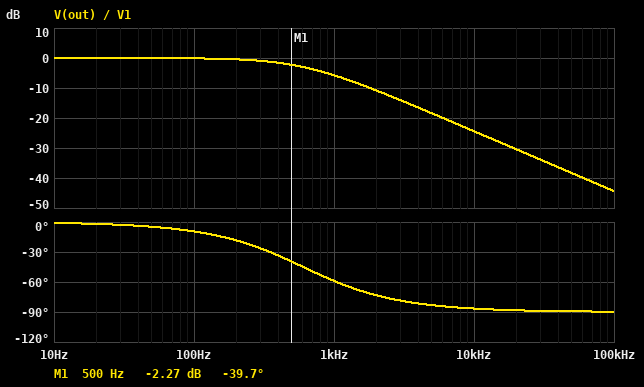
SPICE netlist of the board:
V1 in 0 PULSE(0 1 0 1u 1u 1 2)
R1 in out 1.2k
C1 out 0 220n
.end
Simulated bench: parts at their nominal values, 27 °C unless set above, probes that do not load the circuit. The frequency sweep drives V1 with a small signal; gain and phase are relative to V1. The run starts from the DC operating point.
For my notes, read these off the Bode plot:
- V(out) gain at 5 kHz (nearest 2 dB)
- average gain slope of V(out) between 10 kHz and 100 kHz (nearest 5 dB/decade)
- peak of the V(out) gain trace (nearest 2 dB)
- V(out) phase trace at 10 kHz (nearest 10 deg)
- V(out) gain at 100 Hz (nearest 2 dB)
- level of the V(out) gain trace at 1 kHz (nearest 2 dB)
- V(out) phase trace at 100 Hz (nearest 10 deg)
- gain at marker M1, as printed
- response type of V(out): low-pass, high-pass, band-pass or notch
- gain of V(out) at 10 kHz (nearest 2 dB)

-18 dB
-20 dB/decade
0 dB
-90 deg
0 dB
-6 dB
-10 deg
-2.27 dB
low-pass
-24 dB
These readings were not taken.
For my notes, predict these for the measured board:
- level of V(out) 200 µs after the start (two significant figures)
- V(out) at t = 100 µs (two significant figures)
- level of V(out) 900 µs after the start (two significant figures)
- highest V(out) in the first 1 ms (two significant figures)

530 mV
310 mV
970 mV
980 mV
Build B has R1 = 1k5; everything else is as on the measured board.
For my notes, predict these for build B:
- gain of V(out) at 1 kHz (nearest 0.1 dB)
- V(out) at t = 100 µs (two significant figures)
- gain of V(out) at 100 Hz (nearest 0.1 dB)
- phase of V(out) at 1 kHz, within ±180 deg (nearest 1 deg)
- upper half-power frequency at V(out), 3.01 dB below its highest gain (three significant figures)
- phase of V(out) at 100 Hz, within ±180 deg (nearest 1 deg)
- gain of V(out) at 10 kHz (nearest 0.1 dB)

-7.2 dB
260 mV
-0.2 dB
-64 deg
482 Hz
-12 deg
-26.3 dB
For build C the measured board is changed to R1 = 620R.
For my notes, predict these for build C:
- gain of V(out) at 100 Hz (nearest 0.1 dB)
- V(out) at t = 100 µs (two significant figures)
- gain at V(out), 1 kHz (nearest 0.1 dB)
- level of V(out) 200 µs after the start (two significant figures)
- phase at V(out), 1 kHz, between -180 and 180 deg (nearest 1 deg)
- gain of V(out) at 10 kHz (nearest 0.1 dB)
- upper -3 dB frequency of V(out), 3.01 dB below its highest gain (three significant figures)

0 dB
520 mV
-2.4 dB
770 mV
-41 deg
-18.7 dB
1.17 kHz
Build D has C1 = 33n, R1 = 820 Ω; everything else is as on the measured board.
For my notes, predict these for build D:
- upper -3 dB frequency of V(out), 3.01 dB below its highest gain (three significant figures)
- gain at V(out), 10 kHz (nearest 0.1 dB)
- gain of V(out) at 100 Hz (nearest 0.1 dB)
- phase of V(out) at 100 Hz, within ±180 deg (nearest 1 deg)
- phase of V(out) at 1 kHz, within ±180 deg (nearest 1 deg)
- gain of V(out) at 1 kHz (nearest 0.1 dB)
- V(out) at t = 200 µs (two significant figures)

5.88 kHz
-5.9 dB
0 dB
-1 deg
-10 deg
-0.1 dB
1.0 V
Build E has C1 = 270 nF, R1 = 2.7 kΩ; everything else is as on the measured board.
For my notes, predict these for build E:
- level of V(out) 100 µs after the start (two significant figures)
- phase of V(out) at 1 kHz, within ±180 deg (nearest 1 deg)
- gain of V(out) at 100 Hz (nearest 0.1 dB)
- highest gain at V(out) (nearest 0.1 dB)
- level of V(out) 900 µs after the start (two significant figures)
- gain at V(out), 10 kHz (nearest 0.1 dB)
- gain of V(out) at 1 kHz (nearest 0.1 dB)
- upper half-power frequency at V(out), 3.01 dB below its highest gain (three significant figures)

130 mV
-78 deg
-0.8 dB
0 dB
710 mV
-33.2 dB
-13.4 dB
218 Hz
